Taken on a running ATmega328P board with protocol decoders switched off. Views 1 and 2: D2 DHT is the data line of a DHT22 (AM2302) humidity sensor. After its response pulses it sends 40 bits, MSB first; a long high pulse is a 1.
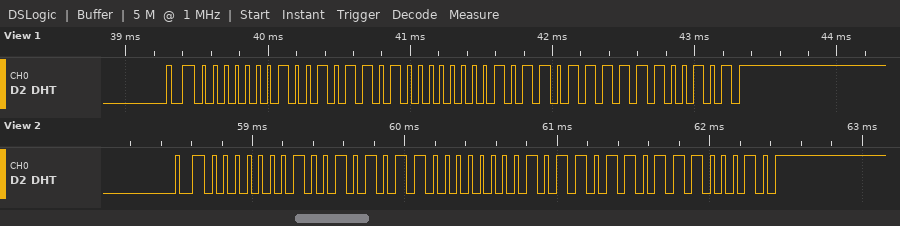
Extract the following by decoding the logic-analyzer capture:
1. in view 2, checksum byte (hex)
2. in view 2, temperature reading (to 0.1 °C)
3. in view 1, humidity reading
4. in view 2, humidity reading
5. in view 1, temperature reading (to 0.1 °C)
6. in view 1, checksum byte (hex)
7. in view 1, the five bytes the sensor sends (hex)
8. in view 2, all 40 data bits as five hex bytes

0xE2
18.2 °C
30.1 %
29.9 %
18.3 °C
0xE5
01 2D 00 B7 E5
01 2B 00 B6 E2
